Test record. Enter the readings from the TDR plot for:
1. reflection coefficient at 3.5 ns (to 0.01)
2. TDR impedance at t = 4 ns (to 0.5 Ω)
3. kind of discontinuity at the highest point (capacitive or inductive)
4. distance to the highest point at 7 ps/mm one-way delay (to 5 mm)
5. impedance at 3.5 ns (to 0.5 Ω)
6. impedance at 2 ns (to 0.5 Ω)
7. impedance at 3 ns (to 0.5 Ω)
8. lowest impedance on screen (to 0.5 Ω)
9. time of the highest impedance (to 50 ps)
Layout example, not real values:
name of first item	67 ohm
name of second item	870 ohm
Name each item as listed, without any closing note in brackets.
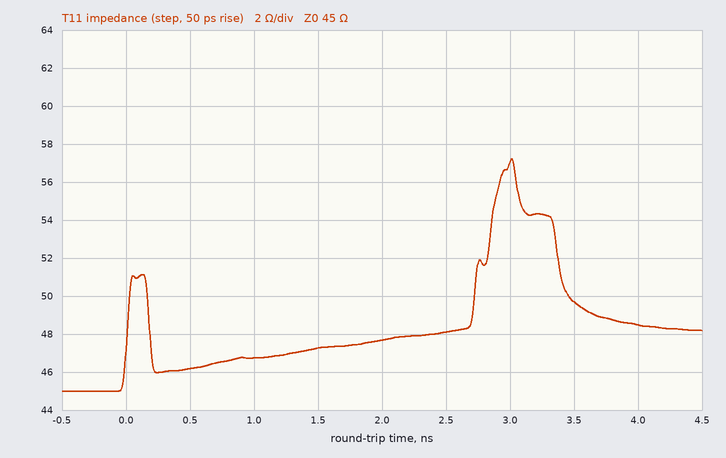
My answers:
reflection coefficient at 3.5 ns	+0.05
TDR impedance at t = 4 ns	48.5 Ω
kind of discontinuity at the highest point	inductive
distance to the highest point at 7 ps/mm one-way delay	215 mm
impedance at 3.5 ns	49.5 Ω
impedance at 2 ns	47.5 Ω
impedance at 3 ns	57.0 Ω
lowest impedance on screen	45.0 Ω
time of the highest impedance	3.00 ns
